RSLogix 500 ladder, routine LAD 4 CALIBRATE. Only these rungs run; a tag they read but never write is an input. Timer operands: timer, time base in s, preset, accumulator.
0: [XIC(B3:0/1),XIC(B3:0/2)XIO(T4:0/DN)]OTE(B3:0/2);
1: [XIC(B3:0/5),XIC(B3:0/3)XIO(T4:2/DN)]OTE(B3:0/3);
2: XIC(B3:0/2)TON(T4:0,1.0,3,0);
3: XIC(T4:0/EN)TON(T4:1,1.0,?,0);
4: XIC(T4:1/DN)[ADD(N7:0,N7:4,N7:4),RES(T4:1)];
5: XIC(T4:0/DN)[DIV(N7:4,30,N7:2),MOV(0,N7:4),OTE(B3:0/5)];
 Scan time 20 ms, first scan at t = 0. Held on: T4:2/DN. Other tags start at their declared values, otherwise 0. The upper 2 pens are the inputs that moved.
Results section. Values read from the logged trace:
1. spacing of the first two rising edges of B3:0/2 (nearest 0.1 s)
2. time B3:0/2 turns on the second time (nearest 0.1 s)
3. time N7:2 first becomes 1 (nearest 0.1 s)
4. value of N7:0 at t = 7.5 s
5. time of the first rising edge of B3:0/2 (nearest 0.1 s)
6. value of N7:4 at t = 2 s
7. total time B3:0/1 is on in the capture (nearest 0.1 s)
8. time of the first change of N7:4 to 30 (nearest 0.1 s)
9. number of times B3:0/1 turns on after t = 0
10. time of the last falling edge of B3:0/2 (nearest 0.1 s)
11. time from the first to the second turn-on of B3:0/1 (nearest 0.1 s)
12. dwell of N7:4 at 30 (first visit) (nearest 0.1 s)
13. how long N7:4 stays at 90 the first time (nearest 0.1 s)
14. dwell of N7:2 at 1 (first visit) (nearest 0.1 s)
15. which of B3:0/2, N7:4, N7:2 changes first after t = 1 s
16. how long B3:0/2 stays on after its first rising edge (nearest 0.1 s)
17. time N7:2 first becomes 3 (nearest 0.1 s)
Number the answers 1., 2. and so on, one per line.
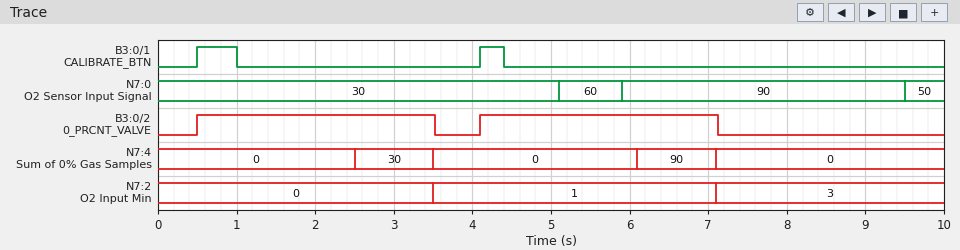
1. 3.6 s
2. 4.1 s
3. 3.5 s
4. 90
5. 0.5 s
6. 0
7. 0.8 s
8. 2.5 s
9. 2
10. 7.1 s
11. 3.6 s
12. 1.0 s
13. 1.0 s
14. 3.6 s
15. N7:4
16. 3.0 s
17. 7.1 s
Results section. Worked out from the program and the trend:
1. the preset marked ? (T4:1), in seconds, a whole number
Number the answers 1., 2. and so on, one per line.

1. 2 s
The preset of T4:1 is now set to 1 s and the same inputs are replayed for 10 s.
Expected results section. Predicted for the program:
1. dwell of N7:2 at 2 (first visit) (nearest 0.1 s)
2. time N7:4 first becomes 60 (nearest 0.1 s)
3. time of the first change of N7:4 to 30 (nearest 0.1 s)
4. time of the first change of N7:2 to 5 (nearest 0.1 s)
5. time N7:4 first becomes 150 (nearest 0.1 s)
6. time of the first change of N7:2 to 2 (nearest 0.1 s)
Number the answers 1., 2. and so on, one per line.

1. 3.6 s
2. 2.5 s
3. 1.5 s
4. 7.1 s
5. 6.1 s
6. 3.5 s
